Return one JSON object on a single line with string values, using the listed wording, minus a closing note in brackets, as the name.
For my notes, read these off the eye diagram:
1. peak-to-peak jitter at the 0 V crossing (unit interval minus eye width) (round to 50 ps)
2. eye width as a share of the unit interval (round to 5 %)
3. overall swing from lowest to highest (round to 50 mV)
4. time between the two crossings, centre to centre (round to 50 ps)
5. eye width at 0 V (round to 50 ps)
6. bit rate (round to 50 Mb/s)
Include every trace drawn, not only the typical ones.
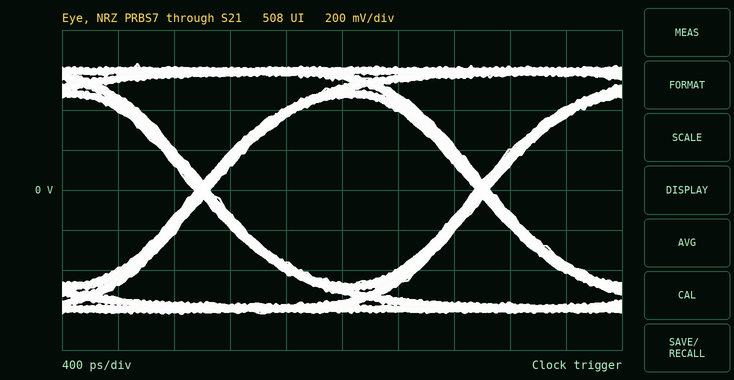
{"peak-to-peak jitter at the 0 V crossing (unit interval minus eye width)": "100 ps", "eye width as a share of the unit interval": "95 %", "overall swing from lowest to highest": "1.25 V", "time between the two crossings, centre to centre": "2.00 ns", "eye width at 0 V": "1.90 ns", "bit rate": "500 Mb/s"}
